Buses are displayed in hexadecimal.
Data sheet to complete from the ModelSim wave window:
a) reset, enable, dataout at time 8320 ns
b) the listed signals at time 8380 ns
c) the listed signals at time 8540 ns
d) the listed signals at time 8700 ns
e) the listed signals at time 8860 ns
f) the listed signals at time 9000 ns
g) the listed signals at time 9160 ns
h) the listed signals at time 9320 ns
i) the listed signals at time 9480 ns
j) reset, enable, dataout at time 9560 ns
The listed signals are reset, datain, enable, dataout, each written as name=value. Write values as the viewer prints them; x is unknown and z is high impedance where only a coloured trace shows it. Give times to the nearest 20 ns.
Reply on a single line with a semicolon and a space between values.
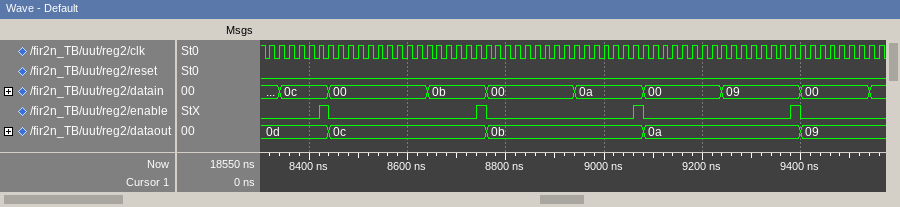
reset=0, enable=0, dataout=0d; reset=0, datain=0c, enable=0, dataout=0d; reset=0, datain=00, enable=0, dataout=0c; reset=0, datain=0b, enable=0, dataout=0c; reset=0, datain=00, enable=0, dataout=0b; reset=0, datain=0a, enable=0, dataout=0b; reset=0, datain=00, enable=0, dataout=0a; reset=0, datain=09, enable=0, dataout=0a; reset=0, datain=00, enable=0, dataout=09; reset=0, enable=0, dataout=09
